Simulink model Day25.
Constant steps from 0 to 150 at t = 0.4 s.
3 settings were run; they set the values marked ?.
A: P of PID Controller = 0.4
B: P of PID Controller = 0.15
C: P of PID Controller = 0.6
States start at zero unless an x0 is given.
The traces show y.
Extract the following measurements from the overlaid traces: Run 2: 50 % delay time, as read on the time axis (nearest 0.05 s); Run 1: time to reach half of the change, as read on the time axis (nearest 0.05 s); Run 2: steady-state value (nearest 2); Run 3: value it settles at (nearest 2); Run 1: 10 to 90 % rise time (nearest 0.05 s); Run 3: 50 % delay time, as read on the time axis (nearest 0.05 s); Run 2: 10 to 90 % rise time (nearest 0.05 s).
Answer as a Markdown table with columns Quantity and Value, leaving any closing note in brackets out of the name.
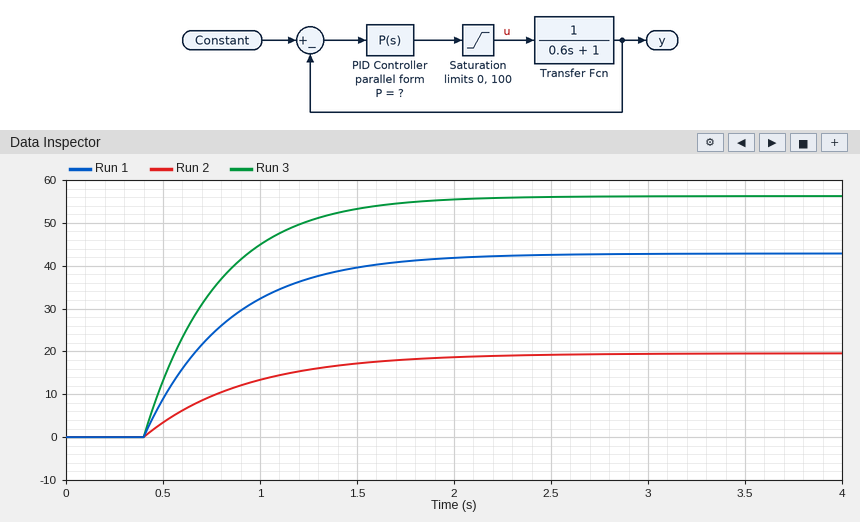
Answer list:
| Quantity | Value |
|---|---|
| Run 2: 50 % delay time, as read on the time axis | 0.75 s |
| Run 1: time to reach half of the change, as read on the time axis | 0.70 s |
| Run 2: steady-state value | 20 |
| Run 3: value it settles at | 56 |
| Run 1: 10 to 90 % rise time | 0.95 s |
| Run 3: 50 % delay time, as read on the time axis | 0.65 s |
| Run 2: 10 to 90 % rise time | 1.15 s |
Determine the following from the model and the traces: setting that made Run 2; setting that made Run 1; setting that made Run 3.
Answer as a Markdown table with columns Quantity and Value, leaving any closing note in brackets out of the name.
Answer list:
| Quantity | Value |
|---|---|
| setting that made Run 2 | B |
| setting that made Run 1 | A |
| setting that made Run 3 | C |
